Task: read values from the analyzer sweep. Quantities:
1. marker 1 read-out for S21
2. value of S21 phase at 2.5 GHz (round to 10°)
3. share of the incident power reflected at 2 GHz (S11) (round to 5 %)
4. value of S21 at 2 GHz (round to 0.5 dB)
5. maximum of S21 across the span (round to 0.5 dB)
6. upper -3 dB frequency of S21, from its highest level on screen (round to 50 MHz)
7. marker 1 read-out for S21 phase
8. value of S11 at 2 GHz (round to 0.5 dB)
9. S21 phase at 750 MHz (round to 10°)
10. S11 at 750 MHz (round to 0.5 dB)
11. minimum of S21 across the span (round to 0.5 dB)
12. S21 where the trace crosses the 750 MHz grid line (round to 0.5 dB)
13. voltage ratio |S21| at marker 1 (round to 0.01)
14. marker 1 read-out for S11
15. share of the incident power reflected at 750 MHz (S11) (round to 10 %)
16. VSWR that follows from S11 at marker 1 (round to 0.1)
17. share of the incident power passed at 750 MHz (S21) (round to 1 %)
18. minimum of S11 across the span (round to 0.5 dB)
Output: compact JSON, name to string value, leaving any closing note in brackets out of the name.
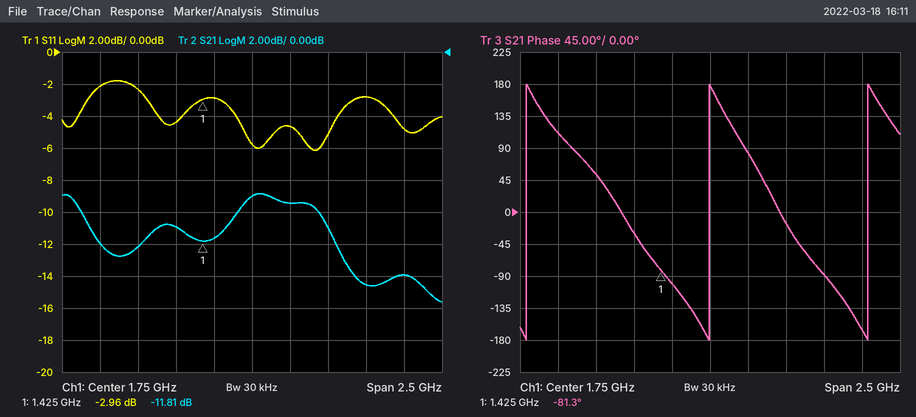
{"marker 1 read-out for S21": "-11.81 dB", "value of S21 phase at 2.5 GHz": "-90°", "share of the incident power reflected at 2 GHz (S11)": "35 %", "value of S21 at 2 GHz": "-9.5 dB", "maximum of S21 across the span": "-9.0 dB", "upper -3 dB frequency of S21, from its highest level on screen": "2.30 GHz", "marker 1 read-out for S21 phase": "-81.3°", "value of S11 at 2 GHz": "-4.5 dB", "S21 phase at 750 MHz": "110°", "S11 at 750 MHz": "-2.0 dB", "minimum of S21 across the span": "-15.5 dB", "S21 where the trace crosses the 750 MHz grid line": "-12.0 dB", "voltage ratio |S21| at marker 1": "0.26", "marker 1 read-out for S11": "-2.96 dB", "share of the incident power reflected at 750 MHz (S11)": "60 %", "VSWR that follows from S11 at marker 1": "5.9", "share of the incident power passed at 750 MHz (S21)": "6 %", "minimum of S11 across the span": "-6.0 dB"}
